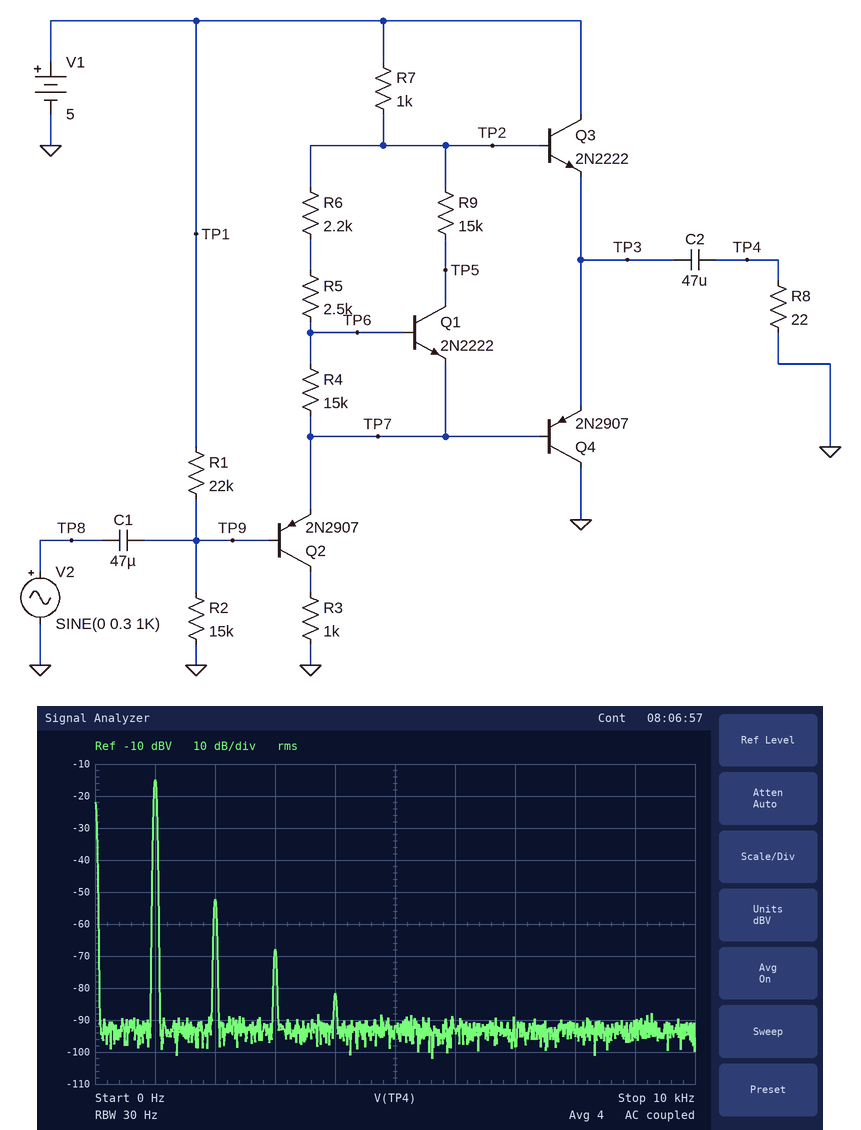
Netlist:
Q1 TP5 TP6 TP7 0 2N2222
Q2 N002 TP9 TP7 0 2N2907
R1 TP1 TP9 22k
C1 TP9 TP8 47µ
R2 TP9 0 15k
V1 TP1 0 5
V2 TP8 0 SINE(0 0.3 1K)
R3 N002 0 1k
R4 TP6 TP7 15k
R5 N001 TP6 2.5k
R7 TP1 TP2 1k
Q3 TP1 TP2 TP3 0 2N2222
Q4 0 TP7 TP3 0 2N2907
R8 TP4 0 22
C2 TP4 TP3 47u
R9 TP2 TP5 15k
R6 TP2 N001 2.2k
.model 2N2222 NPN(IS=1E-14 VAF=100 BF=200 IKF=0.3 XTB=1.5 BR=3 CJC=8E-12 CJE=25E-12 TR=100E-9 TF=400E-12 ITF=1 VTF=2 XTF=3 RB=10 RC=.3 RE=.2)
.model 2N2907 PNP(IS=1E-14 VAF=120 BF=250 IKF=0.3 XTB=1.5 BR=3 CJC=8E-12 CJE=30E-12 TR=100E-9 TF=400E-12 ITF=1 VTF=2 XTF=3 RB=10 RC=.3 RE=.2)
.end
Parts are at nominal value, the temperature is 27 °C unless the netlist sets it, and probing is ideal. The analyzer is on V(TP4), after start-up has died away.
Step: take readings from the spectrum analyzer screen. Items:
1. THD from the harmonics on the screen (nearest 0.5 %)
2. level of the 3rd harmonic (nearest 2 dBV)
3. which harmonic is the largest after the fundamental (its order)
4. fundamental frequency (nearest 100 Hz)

1.5 %
-68 dBV
2
1.0 kHz
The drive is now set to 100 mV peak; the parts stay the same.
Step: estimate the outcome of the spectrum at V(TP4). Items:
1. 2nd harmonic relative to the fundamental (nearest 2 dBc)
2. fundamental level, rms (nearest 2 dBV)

-48 dBc
-24 dBV
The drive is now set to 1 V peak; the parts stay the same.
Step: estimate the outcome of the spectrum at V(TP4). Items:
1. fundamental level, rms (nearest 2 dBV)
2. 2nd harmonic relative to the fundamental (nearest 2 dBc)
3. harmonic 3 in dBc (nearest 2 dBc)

-6 dBV
-16 dBc
-24 dBc
